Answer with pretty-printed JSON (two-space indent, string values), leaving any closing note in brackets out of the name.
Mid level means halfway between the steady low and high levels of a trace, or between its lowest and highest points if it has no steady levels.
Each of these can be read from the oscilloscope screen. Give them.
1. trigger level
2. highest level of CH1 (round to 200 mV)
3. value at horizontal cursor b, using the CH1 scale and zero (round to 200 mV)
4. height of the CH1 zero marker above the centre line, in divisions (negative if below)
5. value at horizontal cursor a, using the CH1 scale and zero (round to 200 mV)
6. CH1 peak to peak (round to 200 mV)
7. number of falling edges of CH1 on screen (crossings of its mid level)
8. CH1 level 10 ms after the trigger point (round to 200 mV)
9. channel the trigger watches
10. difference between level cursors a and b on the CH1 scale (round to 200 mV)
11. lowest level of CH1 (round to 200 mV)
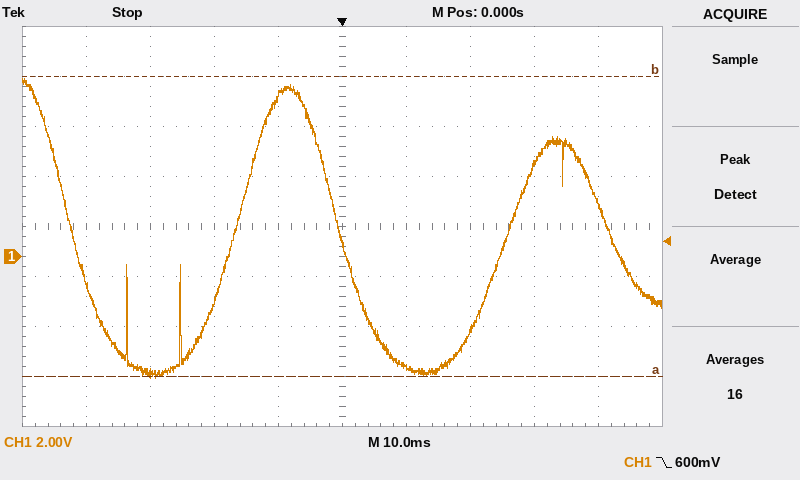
{
  "trigger level": "600 mV",
  "highest level of CH1": "7.2 V",
  "value at horizontal cursor b, using the CH1 scale and zero": "7.2 V",
  "height of the CH1 zero marker above the centre line, in divisions": "-0.6 div",
  "value at horizontal cursor a, using the CH1 scale and zero": "-4.8 V",
  "CH1 peak to peak": "12.0 V",
  "number of falling edges of CH1 on screen": "3",
  "CH1 level 10 ms after the trigger point": "-4.4 V",
  "channel the trigger watches": "CH1",
  "difference between level cursors a and b on the CH1 scale": "12.0 V",
  "lowest level of CH1": "-4.8 V"
}
